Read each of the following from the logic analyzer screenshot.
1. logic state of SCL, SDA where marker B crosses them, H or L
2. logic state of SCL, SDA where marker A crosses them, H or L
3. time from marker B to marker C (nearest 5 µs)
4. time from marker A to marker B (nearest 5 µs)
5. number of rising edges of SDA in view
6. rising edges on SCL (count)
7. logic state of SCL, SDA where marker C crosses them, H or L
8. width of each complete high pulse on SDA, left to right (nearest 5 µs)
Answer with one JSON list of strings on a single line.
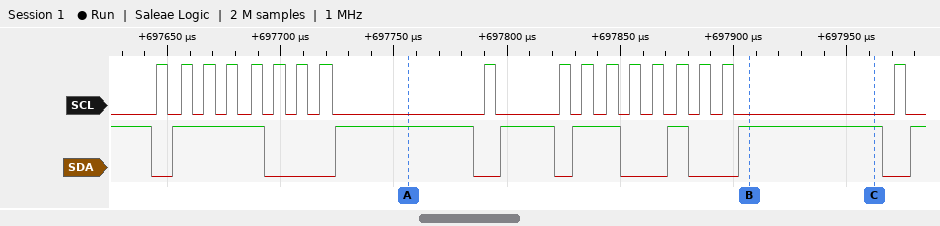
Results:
["SCL=L, SDA=H", "SCL=L, SDA=H", "55 µs", "150 µs", "7", "18", "SCL=L, SDA=H", "40 µs, 60 µs, 25 µs, 20 µs, 10 µs, 65 µs"]
